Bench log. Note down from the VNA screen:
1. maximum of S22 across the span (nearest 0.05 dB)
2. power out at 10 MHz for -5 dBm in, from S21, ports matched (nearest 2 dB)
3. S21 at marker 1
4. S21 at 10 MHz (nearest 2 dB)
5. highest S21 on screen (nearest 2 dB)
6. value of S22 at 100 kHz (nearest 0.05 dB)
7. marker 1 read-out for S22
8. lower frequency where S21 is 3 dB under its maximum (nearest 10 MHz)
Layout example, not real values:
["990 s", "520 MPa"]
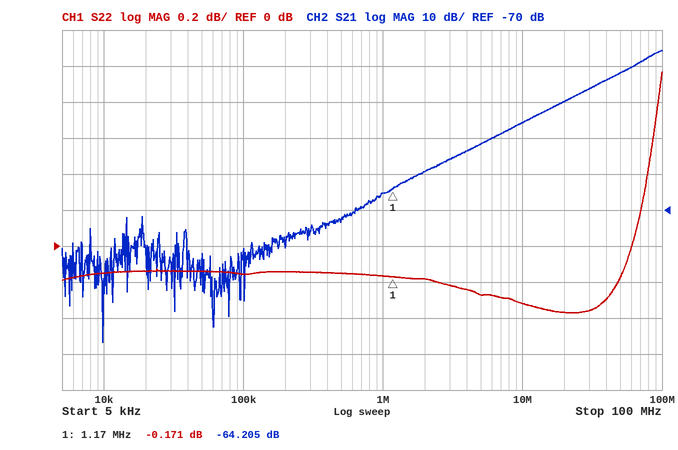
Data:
["0.95 dB", "-50 dBm", "-64.205 dB", "-46 dB", "-26 dB", "-0.15 dB", "-0.171 dB", "70 MHz"]
